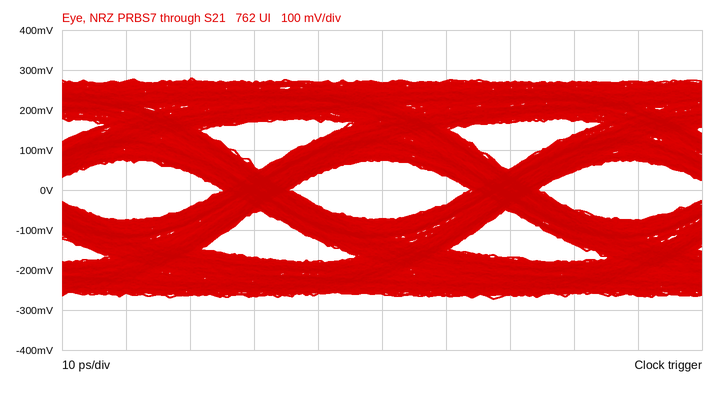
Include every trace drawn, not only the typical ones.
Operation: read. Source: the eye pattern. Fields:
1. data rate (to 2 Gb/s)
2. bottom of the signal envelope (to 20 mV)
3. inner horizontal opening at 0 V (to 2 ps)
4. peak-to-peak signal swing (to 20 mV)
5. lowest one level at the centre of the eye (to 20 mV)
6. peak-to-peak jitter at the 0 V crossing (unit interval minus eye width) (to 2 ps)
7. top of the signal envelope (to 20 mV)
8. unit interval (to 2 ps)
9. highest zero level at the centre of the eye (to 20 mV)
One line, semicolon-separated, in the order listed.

26 Gb/s; -280 mV; 28 ps; 560 mV; 80 mV; 10 ps; 280 mV; 38 ps; -80 mV
